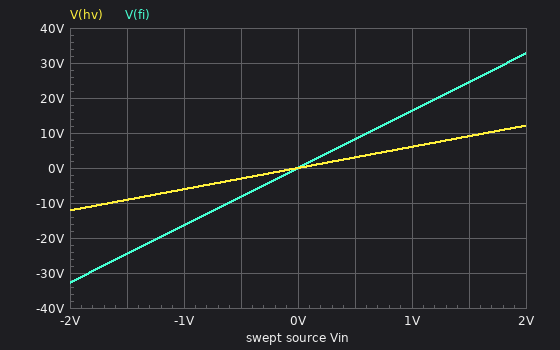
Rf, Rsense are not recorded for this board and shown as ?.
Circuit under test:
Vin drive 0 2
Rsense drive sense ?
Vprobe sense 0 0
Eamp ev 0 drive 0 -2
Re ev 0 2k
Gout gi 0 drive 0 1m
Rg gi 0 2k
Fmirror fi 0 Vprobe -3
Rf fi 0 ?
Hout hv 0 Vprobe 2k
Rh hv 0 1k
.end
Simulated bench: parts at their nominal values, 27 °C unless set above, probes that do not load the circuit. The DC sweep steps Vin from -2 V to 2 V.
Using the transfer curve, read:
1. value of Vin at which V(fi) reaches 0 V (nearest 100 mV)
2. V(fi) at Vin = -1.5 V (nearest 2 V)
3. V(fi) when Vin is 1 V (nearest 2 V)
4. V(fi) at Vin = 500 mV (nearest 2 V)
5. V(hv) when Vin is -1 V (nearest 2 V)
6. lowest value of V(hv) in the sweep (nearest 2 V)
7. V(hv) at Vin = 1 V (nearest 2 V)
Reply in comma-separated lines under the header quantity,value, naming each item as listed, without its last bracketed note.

quantity,value
value of Vin at which V(fi) reaches 0 V,0 V
V(fi) at Vin = -1.5 V,-24 V
V(fi) when Vin is 1 V,16 V
V(fi) at Vin = 500 mV,8 V
V(hv) when Vin is -1 V,-6 V
lowest value of V(hv) in the sweep,-12 V
V(hv) at Vin = 1 V,6 V
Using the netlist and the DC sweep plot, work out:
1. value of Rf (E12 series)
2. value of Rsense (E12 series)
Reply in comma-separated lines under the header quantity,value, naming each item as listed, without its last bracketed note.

quantity,value
value of Rf,1.8 kΩ
value of Rsense,330 Ω
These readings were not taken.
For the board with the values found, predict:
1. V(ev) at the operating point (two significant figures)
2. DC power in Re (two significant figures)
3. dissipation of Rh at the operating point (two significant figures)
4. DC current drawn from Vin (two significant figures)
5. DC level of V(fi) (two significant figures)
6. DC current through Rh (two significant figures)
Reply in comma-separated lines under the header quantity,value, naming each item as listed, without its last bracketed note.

quantity,value
V(ev) at the operating point,-4.0 V
DC power in Re,8.0 mW
dissipation of Rh at the operating point,150 mW
DC current drawn from Vin,6.1 mA
DC level of V(fi),33 V
DC current through Rh,12 mA
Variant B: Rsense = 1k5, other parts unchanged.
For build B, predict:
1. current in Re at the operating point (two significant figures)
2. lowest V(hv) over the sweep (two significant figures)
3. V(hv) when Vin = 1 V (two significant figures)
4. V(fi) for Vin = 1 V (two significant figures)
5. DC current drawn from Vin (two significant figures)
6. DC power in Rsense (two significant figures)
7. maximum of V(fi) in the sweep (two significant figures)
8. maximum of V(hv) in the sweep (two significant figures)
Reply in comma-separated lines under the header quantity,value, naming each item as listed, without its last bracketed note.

quantity,value
current in Re at the operating point,2.0 mA
lowest V(hv) over the sweep,-2.7 V
V(hv) when Vin = 1 V,1.3 V
V(fi) for Vin = 1 V,3.6 V
DC current drawn from Vin,1.3 mA
DC power in Rsense,2.7 mW
maximum of V(fi) in the sweep,7.2 V
maximum of V(hv) in the sweep,2.7 V
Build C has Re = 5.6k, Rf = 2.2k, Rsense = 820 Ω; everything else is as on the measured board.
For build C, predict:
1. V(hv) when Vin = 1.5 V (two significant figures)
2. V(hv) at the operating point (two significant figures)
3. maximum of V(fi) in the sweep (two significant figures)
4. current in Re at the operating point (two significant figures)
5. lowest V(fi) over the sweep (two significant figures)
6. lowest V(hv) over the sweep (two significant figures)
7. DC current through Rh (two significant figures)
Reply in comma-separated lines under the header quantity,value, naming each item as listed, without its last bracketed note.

quantity,value
V(hv) when Vin = 1.5 V,3.7 V
V(hv) at the operating point,4.9 V
maximum of V(fi) in the sweep,16 V
current in Re at the operating point,710 µA
lowest V(fi) over the sweep,-16 V
lowest V(hv) over the sweep,-4.9 V
DC current through Rh,4.9 mA
